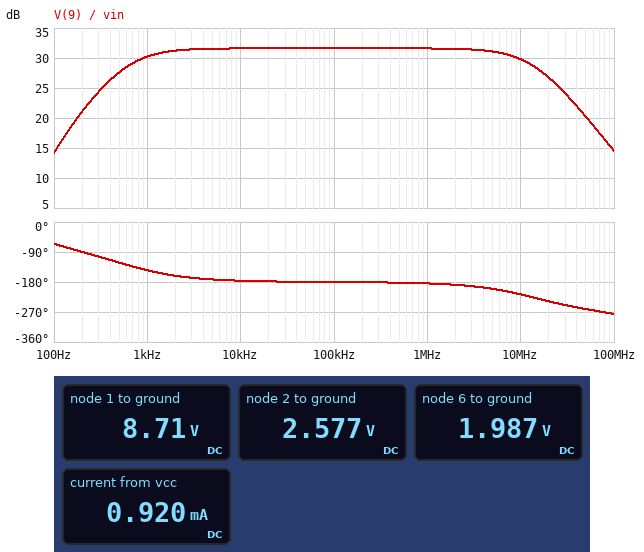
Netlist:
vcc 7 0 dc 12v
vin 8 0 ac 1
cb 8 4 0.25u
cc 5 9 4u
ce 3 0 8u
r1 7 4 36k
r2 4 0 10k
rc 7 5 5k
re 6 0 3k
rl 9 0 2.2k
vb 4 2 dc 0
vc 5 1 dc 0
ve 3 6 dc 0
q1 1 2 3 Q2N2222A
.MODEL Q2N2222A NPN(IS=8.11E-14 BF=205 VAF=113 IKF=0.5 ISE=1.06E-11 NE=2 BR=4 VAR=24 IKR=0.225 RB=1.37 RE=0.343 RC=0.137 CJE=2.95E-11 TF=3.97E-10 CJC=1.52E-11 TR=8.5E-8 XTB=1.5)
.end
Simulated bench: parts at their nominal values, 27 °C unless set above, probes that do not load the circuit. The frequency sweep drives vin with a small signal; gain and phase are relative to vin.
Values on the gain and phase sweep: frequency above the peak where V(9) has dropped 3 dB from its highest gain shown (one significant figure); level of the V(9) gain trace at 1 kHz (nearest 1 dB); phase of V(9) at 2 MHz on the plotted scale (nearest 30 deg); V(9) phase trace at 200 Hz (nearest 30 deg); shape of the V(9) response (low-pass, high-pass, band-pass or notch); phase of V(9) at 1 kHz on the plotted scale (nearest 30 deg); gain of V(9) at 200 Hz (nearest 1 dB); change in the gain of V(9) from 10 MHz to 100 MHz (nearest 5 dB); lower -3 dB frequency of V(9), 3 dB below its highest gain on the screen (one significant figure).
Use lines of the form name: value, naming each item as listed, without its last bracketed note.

frequency above the peak where V(9) has dropped 3 dB from its highest gain shown: 10 MHz
level of the V(9) gain trace at 1 kHz: 30 dB
phase of V(9) at 2 MHz on the plotted scale: -180 deg
V(9) phase trace at 200 Hz: -90 deg
shape of the V(9) response: band-pass
phase of V(9) at 1 kHz on the plotted scale: -150 deg
gain of V(9) at 200 Hz: 21 dB
change in the gain of V(9) from 10 MHz to 100 MHz: -15 dB
lower -3 dB frequency of V(9), 3 dB below its highest gain on the screen: 600 Hz
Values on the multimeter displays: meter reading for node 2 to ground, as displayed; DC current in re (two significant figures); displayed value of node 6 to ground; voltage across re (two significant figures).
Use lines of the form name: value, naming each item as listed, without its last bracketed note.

meter reading for node 2 to ground, as displayed: 2.577 V
DC current in re: 660 µA
displayed value of node 6 to ground: 1.987 V
voltage across re: 2.0 V
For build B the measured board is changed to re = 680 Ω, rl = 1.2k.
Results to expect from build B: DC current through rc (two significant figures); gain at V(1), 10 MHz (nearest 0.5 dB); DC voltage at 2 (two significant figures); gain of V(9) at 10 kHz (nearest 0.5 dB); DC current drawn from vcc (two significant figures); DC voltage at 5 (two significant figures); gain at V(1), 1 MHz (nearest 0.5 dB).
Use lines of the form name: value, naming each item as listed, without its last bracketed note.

DC current through rc: 2.1 mA
gain at V(1), 10 MHz: 5.0 dB
DC voltage at 2: 2.1 V
gain of V(9) at 10 kHz: 13.5 dB
DC current drawn from vcc: 2.4 mA
DC voltage at 5: 1.5 V
gain at V(1), 1 MHz: 16.0 dB
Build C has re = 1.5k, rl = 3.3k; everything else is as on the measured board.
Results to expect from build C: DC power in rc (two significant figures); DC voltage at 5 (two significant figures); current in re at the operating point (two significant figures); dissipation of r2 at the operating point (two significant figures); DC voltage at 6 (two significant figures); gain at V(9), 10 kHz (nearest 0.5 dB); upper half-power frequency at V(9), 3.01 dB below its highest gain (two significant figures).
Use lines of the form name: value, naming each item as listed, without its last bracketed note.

DC power in rc: 8.3 mW
DC voltage at 5: 5.6 V
current in re at the operating point: 1.3 mA
dissipation of r2 at the operating point: 650 µW
DC voltage at 6: 1.9 V
gain at V(9), 10 kHz: 39.5 dB
upper half-power frequency at V(9), 3.01 dB below its highest gain: 8.6 MHz
